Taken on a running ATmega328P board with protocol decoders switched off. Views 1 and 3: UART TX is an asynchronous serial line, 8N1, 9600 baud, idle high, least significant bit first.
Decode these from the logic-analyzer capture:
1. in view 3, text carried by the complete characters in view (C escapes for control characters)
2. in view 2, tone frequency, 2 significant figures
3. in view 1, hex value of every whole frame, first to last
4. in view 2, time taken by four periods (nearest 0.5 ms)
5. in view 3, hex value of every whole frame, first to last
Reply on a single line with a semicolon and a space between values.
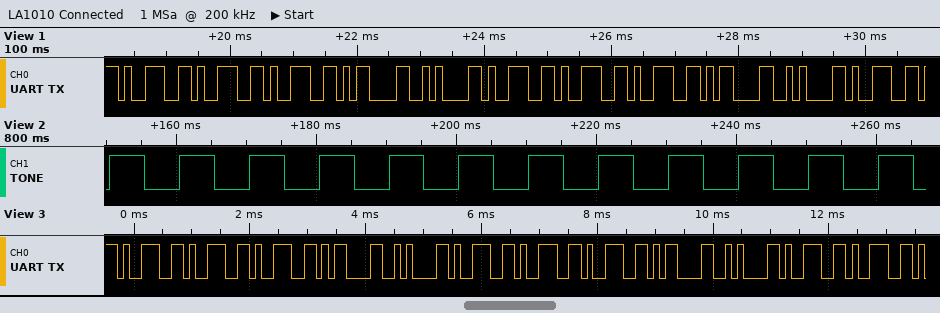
"999\r\n999\r\n99"; 100 Hz; 39 39 39 0D 0A 39 39 39 0D 0A 39; 40.0 ms; 39 39 39 0D 0A 39 39 39 0D 0A 39 39
